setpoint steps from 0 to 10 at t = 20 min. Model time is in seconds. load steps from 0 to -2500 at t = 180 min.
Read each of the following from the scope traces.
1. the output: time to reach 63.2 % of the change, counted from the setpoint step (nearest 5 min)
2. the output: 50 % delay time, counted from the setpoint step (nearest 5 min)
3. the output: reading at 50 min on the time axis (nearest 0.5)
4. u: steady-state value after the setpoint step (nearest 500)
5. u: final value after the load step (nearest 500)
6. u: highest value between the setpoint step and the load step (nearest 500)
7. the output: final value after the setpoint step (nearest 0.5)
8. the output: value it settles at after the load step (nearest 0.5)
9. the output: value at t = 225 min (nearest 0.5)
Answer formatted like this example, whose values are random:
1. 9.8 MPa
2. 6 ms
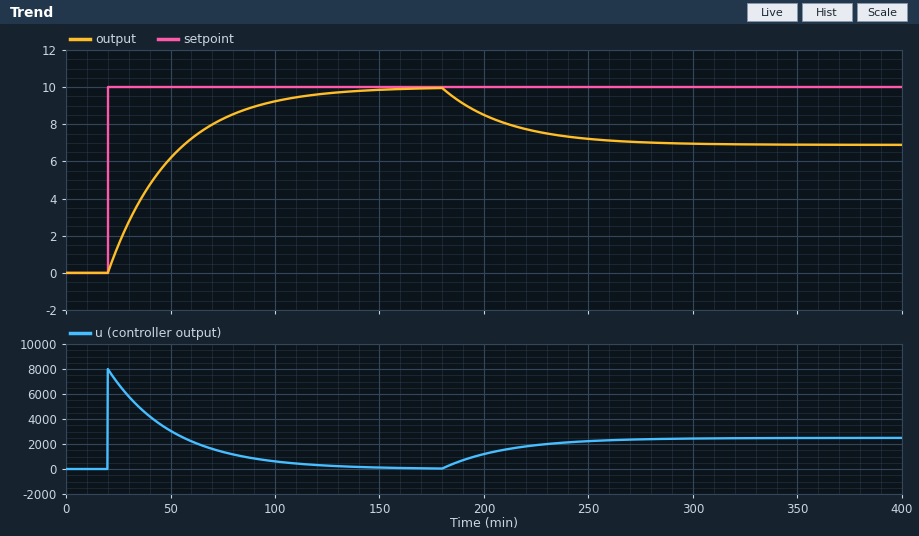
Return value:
1. 30 min
2. 20 min
3. 6.0
4. 0
5. 2500
6. 8000
7. 10.0
8. 7.0
9. 7.5
